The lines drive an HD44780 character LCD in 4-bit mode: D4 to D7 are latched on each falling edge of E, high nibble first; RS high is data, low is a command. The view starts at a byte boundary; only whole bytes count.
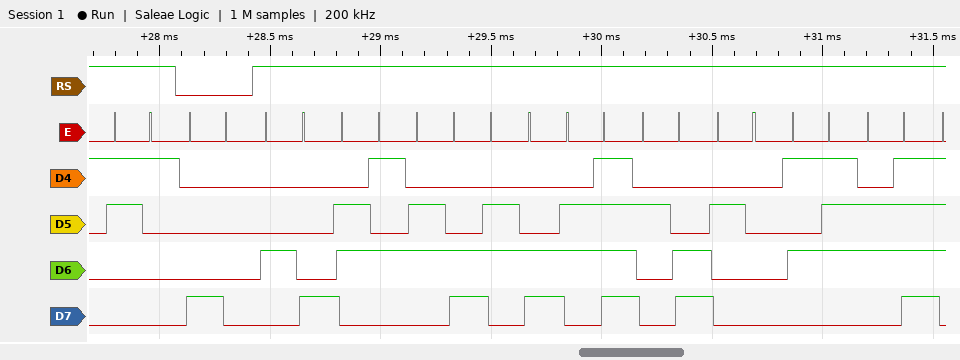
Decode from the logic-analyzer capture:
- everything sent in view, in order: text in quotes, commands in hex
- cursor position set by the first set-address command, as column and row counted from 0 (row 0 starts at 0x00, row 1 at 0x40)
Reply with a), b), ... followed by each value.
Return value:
a) "1" 0x80 "Hello, Wo"
b) column 0, row 0
